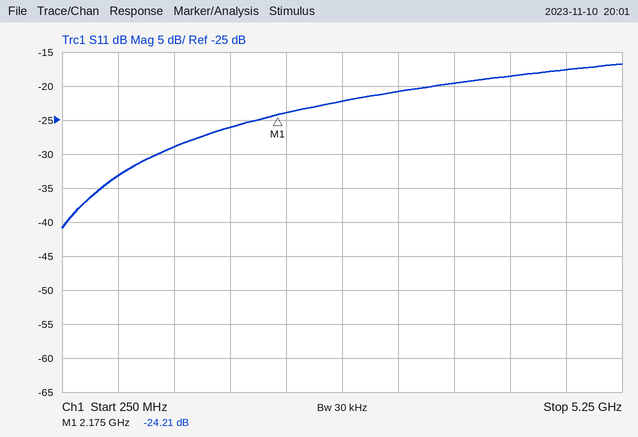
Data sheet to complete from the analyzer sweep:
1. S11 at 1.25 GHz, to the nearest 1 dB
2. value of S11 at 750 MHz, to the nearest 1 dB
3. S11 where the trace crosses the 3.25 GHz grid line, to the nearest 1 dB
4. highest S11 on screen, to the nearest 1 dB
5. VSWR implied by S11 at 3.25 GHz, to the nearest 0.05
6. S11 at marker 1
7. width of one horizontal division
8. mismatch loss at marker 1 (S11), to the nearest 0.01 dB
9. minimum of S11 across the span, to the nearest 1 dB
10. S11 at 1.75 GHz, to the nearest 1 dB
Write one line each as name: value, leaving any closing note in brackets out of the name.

S11 at 1.25 GHz, to the nearest 1 dB: -29 dB
value of S11 at 750 MHz, to the nearest 1 dB: -33 dB
S11 where the trace crosses the 3.25 GHz grid line, to the nearest 1 dB: -21 dB
highest S11 on screen, to the nearest 1 dB: -17 dB
VSWR implied by S11 at 3.25 GHz, to the nearest 0.05: 1.20
S11 at marker 1: -24.21 dB
width of one horizontal division: 500 MHz
mismatch loss at marker 1 (S11), to the nearest 0.01 dB: 0.02 dB
minimum of S11 across the span, to the nearest 1 dB: -41 dB
S11 at 1.75 GHz, to the nearest 1 dB: -26 dB
